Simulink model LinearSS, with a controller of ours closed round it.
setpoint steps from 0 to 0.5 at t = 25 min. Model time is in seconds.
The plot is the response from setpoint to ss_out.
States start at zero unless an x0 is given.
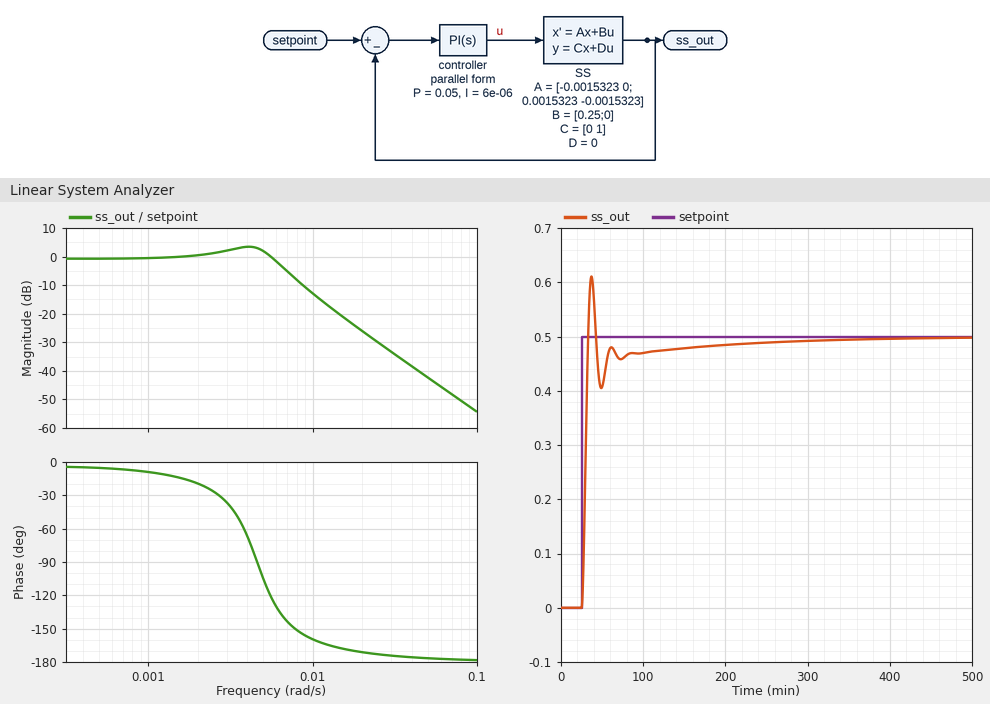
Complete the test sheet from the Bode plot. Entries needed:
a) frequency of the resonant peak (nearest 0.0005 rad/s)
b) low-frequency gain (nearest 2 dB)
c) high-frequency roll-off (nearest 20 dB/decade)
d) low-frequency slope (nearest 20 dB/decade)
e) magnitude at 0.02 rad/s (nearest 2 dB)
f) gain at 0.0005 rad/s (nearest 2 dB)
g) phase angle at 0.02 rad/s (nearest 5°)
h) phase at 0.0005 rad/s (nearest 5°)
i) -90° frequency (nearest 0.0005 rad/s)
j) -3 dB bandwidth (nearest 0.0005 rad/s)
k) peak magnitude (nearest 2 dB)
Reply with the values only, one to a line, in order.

0.0040 rad/s
0 dB
-40 dB/decade
0 dB/decade
-26 dB
0 dB
-170°
-5°
0.0045 rad/s
0.0065 rad/s
4 dB
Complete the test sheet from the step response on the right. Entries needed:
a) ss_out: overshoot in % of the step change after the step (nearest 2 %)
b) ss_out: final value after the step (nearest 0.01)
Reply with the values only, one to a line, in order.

22 %
0.50
